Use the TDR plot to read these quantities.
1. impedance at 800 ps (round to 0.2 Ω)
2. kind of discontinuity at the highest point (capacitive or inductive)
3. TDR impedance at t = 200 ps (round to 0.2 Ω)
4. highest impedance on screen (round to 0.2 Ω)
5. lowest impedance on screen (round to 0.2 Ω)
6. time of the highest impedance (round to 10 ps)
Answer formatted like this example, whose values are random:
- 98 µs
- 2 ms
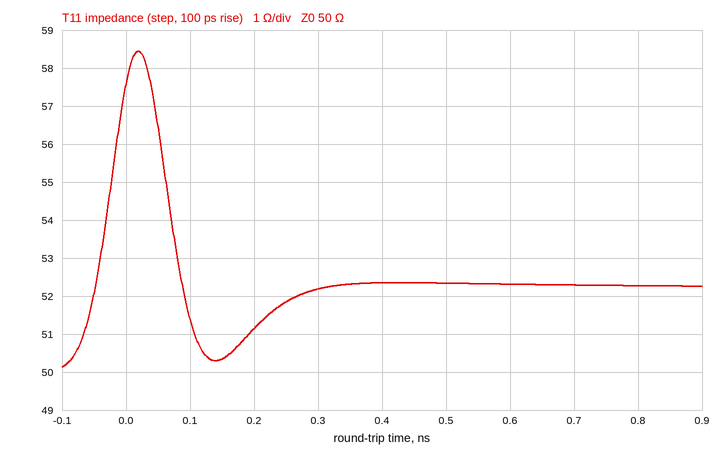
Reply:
- 52.2 Ω
- inductive
- 51.2 Ω
- 58.4 Ω
- 50.2 Ω
- 20 ps
